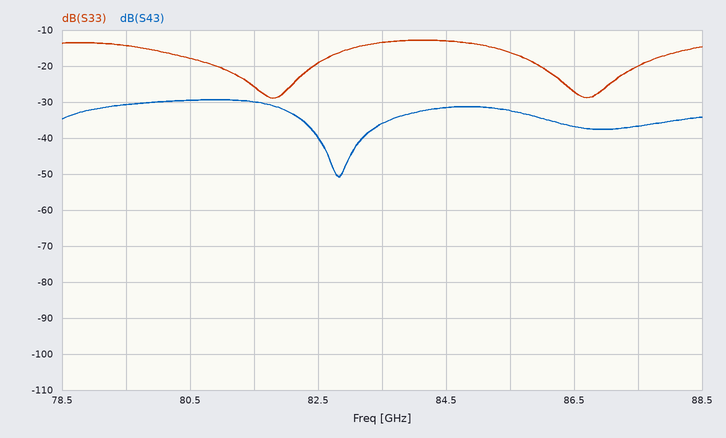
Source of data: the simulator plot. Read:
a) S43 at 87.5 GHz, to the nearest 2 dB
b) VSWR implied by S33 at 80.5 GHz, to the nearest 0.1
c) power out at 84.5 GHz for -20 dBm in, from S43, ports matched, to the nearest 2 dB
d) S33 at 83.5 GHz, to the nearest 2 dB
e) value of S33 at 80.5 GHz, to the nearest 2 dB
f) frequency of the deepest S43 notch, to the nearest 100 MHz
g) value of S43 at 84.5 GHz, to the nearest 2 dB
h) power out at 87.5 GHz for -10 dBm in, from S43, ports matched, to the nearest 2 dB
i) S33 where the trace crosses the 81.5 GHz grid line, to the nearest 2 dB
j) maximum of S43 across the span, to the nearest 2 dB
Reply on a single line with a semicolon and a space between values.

-36 dB; 1.3; -52 dBm; -14 dB; -18 dB; 82.8 GHz; -32 dB; -46 dBm; -26 dB; -30 dB
